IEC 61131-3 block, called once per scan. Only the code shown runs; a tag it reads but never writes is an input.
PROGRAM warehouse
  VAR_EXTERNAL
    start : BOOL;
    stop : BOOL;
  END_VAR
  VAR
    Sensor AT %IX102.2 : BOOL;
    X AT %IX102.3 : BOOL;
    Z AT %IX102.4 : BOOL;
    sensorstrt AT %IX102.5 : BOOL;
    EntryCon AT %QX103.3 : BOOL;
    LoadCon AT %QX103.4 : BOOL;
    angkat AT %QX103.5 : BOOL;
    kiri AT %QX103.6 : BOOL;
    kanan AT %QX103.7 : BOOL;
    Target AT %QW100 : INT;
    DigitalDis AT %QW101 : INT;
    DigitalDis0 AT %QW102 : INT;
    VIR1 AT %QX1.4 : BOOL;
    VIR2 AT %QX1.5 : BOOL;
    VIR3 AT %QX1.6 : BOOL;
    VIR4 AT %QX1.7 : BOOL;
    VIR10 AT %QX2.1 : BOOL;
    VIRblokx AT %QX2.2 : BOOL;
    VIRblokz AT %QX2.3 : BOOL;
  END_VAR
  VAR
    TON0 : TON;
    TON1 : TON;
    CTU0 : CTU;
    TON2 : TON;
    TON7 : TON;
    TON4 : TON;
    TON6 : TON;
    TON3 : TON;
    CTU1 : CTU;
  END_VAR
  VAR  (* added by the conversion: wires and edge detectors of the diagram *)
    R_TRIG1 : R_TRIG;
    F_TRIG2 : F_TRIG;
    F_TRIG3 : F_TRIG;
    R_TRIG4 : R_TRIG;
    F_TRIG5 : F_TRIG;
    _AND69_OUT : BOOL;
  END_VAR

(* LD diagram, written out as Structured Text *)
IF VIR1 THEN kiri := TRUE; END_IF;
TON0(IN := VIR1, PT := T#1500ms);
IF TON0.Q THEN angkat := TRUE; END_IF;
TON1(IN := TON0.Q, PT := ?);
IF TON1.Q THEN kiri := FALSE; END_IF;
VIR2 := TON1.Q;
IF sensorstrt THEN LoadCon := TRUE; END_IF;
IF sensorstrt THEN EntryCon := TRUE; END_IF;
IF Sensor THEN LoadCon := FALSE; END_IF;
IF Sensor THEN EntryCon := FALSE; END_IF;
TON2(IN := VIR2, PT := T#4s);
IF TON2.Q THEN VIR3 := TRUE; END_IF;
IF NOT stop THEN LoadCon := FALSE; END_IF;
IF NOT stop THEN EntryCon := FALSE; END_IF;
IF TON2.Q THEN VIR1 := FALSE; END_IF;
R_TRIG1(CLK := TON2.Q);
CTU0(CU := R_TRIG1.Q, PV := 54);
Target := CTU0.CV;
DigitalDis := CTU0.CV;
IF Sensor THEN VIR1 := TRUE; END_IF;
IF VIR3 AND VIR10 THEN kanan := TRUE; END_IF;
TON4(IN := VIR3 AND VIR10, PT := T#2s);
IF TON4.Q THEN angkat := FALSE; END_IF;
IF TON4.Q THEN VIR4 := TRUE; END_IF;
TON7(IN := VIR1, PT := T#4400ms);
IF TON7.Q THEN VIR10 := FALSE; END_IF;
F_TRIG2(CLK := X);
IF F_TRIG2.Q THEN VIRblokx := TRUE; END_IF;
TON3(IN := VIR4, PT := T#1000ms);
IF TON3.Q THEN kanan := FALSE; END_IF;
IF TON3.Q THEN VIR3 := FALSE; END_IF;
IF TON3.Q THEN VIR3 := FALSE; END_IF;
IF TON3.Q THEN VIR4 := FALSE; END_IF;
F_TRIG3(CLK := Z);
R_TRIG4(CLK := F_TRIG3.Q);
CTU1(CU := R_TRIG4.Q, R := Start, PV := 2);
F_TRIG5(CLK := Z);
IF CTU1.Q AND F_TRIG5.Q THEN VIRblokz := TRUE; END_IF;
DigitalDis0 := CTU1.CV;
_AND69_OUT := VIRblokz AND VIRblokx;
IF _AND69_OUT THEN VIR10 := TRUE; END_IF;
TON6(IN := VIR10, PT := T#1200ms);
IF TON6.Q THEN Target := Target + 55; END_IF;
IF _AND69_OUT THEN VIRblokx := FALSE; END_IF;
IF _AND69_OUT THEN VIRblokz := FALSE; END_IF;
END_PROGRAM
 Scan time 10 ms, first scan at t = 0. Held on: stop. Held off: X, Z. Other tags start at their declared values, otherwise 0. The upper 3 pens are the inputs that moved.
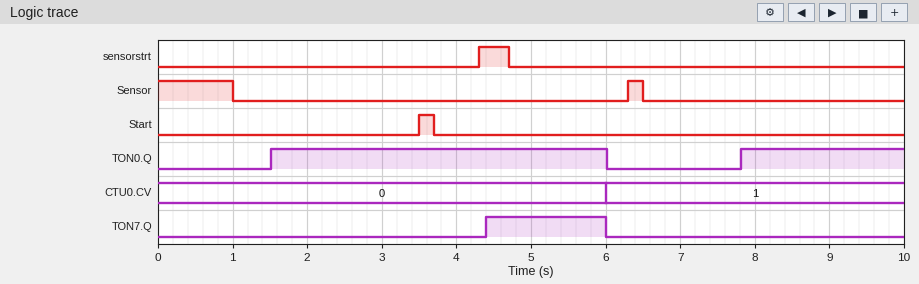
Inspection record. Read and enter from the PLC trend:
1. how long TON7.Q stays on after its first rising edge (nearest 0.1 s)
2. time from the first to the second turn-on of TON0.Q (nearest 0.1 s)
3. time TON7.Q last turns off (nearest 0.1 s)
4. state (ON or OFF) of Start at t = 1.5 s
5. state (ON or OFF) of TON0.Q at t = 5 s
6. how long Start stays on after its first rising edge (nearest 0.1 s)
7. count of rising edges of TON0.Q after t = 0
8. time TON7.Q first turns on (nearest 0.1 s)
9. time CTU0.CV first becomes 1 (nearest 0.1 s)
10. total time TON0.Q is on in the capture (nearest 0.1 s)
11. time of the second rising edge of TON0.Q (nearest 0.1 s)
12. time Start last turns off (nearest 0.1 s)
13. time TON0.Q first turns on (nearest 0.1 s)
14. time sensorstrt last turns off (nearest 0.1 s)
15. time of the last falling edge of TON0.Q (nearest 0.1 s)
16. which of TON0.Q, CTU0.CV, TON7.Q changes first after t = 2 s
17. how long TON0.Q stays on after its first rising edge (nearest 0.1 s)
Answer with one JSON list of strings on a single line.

["1.6 s", "6.3 s", "6.0 s", "OFF", "ON", "0.2 s", "2", "4.4 s", "6.0 s", "6.7 s", "7.8 s", "3.7 s", "1.5 s", "4.7 s", "6.0 s", "TON7.Q", "4.5 s"]
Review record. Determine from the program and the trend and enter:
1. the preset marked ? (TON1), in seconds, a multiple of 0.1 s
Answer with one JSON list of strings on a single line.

["0.5 s"]
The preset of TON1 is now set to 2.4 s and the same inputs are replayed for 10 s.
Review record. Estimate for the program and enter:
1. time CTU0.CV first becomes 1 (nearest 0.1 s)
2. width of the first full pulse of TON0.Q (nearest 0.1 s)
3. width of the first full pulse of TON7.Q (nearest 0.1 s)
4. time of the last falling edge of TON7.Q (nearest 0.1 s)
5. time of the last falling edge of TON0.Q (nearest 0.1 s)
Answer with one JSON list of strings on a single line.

["7.9 s", "6.4 s", "3.5 s", "7.9 s", "7.9 s"]
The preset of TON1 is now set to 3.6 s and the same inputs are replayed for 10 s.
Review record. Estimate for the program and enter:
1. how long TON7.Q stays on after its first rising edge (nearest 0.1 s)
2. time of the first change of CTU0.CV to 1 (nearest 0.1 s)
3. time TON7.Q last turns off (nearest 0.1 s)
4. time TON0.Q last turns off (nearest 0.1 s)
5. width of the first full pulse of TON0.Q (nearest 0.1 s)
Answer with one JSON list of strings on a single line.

["4.7 s", "9.1 s", "9.1 s", "9.1 s", "7.6 s"]
